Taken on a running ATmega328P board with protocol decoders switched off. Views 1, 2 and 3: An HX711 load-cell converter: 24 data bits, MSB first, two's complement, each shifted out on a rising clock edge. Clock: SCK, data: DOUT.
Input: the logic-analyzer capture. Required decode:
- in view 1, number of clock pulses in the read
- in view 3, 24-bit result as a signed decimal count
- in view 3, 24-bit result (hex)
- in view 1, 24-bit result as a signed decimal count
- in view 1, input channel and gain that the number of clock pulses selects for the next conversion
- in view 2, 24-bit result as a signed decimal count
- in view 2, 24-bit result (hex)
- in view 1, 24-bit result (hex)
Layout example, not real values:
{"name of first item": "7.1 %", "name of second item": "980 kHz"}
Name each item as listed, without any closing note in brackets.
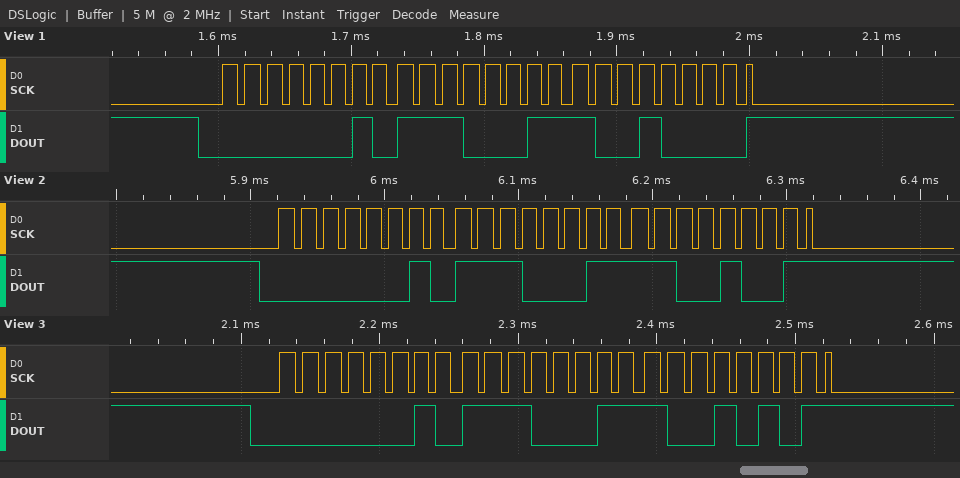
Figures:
{"in view 1, number of clock pulses in the read": "25", "in view 3, 24-bit result as a signed decimal count": "189333", "in view 3, 24-bit result": "0x02E395", "in view 1, 24-bit result as a signed decimal count": "189328", "in view 1, input channel and gain that the number of clock pulses selects for the next conversion": "channel A, gain 128", "in view 2, 24-bit result as a signed decimal count": "189385", "in view 2, 24-bit result": "0x02E3C9", "in view 1, 24-bit result": "0x02E390"}
